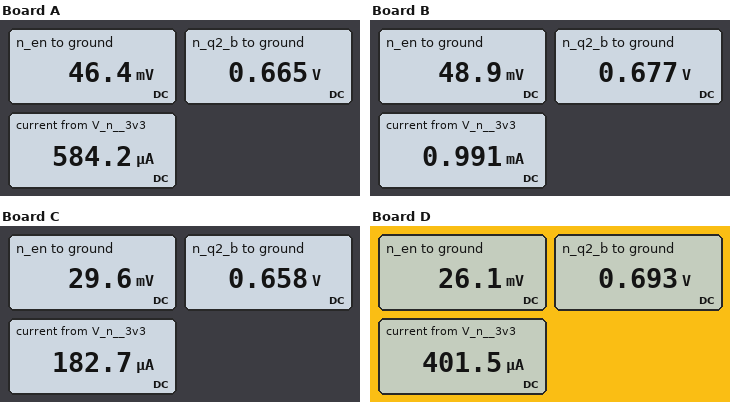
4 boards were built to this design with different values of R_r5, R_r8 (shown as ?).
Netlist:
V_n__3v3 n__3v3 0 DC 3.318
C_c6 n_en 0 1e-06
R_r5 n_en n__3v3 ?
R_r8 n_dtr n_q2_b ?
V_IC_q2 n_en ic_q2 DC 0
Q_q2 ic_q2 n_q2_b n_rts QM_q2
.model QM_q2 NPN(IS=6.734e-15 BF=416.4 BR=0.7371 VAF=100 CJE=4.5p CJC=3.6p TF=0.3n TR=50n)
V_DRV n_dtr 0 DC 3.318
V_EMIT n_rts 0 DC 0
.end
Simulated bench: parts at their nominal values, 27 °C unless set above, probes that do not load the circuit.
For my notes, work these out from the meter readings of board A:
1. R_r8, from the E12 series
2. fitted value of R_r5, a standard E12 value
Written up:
12 kΩ
5.6 kΩ
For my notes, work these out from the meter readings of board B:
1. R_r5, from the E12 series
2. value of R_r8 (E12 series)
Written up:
3.3 kΩ
8.2 kΩ
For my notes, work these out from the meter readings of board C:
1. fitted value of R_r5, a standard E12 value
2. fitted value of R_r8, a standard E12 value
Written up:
18 kΩ
8.2 kΩ
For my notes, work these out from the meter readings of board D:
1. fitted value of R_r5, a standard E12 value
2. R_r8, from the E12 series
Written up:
8.2 kΩ
1.8 kΩ
